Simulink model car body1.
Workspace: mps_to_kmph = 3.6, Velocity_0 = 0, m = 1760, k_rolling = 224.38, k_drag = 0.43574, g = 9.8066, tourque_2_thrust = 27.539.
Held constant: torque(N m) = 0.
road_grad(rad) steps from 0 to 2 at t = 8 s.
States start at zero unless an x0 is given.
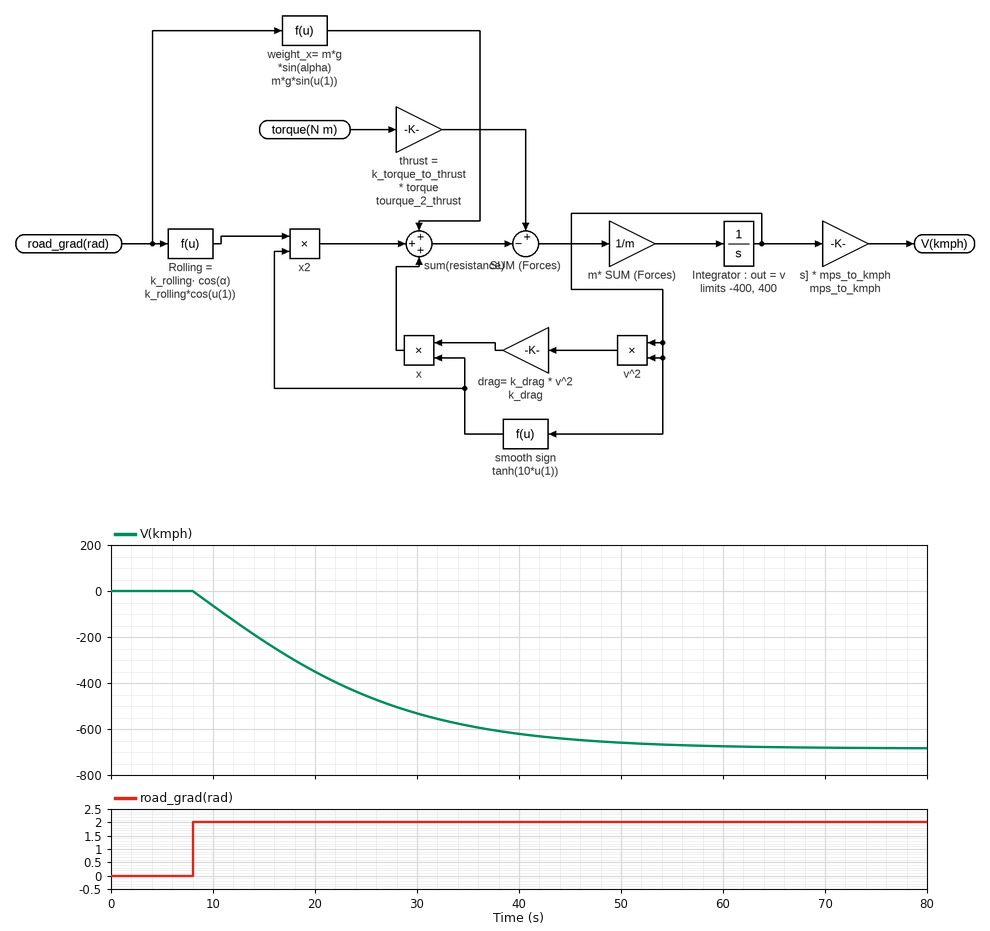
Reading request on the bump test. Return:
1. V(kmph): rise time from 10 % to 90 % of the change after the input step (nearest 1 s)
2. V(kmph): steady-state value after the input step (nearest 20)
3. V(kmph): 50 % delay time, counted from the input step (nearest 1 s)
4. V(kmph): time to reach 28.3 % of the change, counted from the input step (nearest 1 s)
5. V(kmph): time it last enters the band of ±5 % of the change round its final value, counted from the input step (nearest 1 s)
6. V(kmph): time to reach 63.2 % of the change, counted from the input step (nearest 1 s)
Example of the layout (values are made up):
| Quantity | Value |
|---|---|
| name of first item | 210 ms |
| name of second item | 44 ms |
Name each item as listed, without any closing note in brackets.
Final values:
| Quantity | Value |
|---|---|
| V(kmph): rise time from 10 % to 90 % of the change after the input step | 29 s |
| V(kmph): steady-state value after the input step | -680 |
| V(kmph): 50 % delay time, counted from the input step | 12 s |
| V(kmph): time to reach 28.3 % of the change, counted from the input step | 6 s |
| V(kmph): time it last enters the band of ±5 % of the change round its final value, counted from the input step | 39 s |
| V(kmph): time to reach 63.2 % of the change, counted from the input step | 16 s |
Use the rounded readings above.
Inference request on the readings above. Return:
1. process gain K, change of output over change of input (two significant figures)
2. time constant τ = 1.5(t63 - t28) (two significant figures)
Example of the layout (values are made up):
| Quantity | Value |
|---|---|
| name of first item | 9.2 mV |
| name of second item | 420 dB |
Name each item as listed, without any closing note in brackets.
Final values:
| Quantity | Value |
|---|---|
| process gain K, change of output over change of input | -340 |
| time constant τ = 1.5(t63 - t28) | 15 s |
